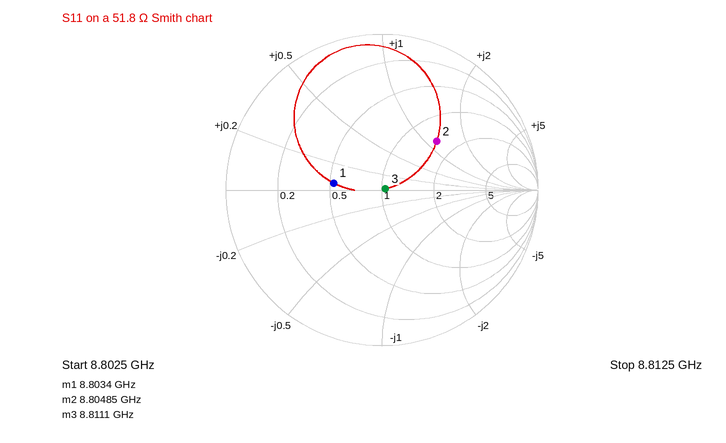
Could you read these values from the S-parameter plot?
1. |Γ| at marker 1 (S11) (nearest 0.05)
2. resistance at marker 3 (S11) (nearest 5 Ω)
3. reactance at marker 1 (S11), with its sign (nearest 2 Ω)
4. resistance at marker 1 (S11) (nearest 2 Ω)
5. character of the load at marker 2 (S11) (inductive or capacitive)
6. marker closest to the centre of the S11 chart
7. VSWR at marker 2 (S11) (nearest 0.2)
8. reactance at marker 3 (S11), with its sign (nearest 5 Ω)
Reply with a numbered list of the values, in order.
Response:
1. 0.30
2. 55 Ω
3. +2 Ω
4. 28 Ω
5. inductive
6. marker 3
7. 2.8
8. 0 Ω
